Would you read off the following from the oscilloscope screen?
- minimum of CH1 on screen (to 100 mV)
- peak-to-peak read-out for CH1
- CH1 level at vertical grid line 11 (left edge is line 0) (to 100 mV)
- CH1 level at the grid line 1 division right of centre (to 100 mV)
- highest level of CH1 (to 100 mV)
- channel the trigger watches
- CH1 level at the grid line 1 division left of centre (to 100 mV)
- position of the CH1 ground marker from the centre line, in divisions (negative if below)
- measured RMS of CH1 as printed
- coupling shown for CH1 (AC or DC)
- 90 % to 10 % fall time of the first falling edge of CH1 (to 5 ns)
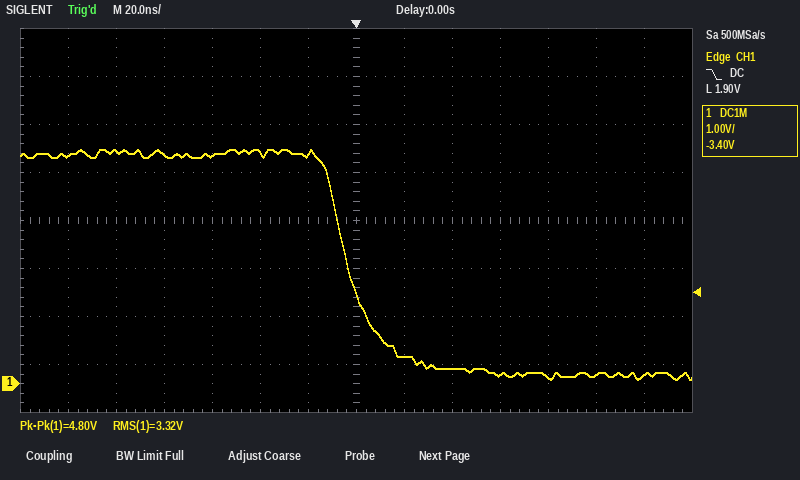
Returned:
100 mV
4.80 V
100 mV
600 mV
4.9 V
CH1
4.8 V
-3.4 div
3.32 V
DC
30 ns
